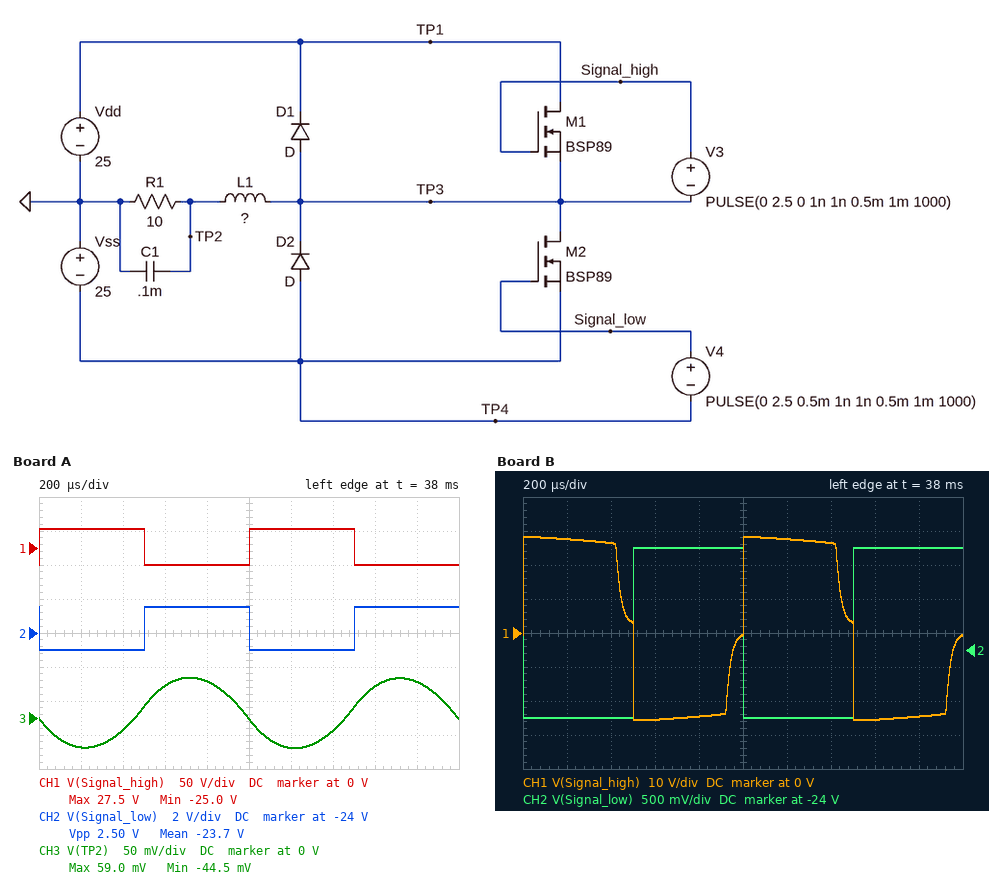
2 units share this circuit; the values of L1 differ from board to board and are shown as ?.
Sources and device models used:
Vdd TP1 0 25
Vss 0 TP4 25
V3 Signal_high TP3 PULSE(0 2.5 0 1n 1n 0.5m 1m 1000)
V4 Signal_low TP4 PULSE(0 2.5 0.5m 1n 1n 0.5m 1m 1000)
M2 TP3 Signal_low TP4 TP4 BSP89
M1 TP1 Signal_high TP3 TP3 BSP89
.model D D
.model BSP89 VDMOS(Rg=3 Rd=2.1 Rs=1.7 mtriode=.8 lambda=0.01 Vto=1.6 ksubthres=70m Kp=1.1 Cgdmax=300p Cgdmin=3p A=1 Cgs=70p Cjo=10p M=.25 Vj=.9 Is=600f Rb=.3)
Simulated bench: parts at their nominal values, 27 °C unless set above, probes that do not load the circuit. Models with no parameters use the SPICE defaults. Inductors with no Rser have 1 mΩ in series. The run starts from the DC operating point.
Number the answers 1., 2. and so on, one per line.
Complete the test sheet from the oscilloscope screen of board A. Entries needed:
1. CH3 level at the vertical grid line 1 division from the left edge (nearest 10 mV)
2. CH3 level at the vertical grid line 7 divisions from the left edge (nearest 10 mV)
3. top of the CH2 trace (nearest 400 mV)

1. -40 mV
2. -20 mV
3. -22.4 V
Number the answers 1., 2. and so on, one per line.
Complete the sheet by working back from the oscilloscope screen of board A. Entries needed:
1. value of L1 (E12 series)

1. 150 mH
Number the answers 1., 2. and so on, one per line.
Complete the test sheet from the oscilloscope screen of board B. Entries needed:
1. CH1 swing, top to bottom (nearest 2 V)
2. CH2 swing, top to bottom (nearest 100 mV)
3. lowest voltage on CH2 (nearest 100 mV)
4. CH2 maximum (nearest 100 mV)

1. 54 V
2. 2.5 V
3. -25.0 V
4. -22.5 V
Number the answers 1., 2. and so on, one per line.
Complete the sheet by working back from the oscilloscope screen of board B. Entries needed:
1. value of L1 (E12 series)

1. 27 mH
